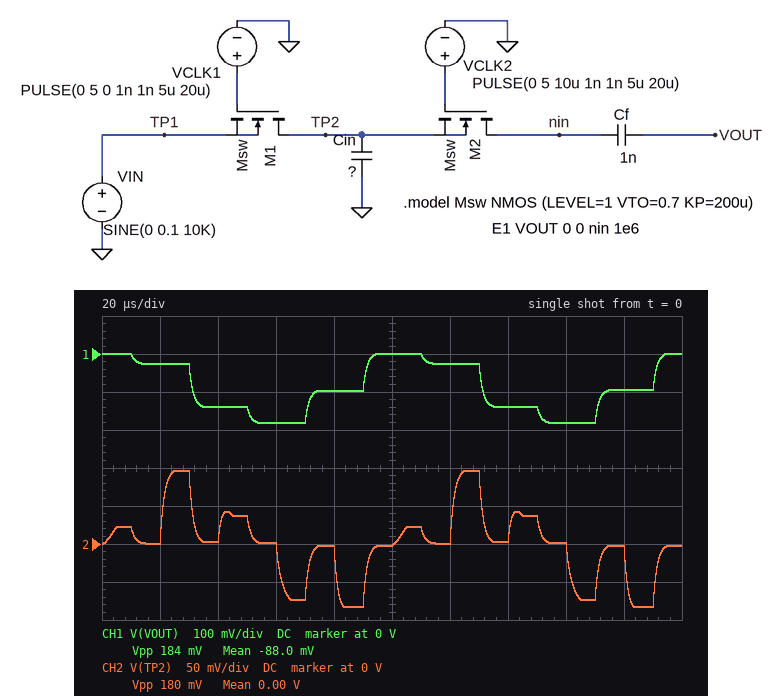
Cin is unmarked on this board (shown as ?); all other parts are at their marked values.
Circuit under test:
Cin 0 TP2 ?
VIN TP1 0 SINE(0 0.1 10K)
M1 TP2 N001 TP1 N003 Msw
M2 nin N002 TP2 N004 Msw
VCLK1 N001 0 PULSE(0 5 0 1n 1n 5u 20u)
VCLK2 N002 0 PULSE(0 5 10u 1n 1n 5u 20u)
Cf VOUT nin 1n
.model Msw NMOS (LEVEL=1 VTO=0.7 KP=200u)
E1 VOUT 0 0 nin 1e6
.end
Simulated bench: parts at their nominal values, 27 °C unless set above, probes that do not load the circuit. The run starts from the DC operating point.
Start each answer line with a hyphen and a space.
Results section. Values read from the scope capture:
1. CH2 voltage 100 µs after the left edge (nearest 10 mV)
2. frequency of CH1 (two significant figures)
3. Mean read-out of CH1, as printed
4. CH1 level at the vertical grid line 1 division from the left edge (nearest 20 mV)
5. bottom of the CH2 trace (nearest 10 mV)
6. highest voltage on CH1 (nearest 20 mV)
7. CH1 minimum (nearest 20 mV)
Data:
- 0 V
- 10 kHz
- -88.0 mV
- -20 mV
- -80 mV
- 0 V
- -180 mV
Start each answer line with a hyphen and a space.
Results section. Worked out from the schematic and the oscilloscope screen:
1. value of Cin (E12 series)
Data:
- 1.2 nF
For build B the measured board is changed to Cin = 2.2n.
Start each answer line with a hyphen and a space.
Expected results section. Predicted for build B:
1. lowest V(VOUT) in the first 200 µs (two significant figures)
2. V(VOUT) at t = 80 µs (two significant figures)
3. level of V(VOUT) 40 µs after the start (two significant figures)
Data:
- -260 mV
- -140 mV
- -190 mV
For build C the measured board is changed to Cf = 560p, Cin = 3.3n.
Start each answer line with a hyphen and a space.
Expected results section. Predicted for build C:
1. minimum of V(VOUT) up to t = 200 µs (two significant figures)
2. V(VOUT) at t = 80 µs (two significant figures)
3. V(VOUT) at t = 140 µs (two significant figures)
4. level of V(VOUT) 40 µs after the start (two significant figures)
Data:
- -520 mV
- -310 mV
- -360 mV
- -370 mV
